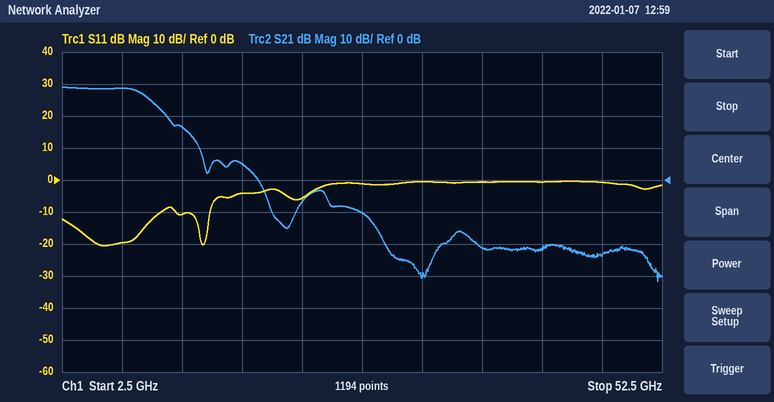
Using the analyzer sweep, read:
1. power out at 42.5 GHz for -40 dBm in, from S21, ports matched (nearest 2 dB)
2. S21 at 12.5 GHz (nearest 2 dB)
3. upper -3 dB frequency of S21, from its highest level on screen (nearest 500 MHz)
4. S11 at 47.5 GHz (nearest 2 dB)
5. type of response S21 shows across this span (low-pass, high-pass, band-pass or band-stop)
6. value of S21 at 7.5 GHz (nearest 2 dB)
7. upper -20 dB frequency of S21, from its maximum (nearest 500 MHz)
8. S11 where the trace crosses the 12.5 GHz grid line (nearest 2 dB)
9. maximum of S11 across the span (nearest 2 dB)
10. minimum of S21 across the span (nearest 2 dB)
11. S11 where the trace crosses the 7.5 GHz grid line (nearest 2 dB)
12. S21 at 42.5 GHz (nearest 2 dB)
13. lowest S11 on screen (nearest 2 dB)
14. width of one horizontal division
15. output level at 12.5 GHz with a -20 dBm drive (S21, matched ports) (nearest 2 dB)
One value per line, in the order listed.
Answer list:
-62 dBm
16 dB
9.5 GHz
0 dB
low-pass
28 dB
14.0 GHz
-10 dB
0 dB
-32 dB
-20 dB
-22 dB
-20 dB
5 GHz
-4 dBm
